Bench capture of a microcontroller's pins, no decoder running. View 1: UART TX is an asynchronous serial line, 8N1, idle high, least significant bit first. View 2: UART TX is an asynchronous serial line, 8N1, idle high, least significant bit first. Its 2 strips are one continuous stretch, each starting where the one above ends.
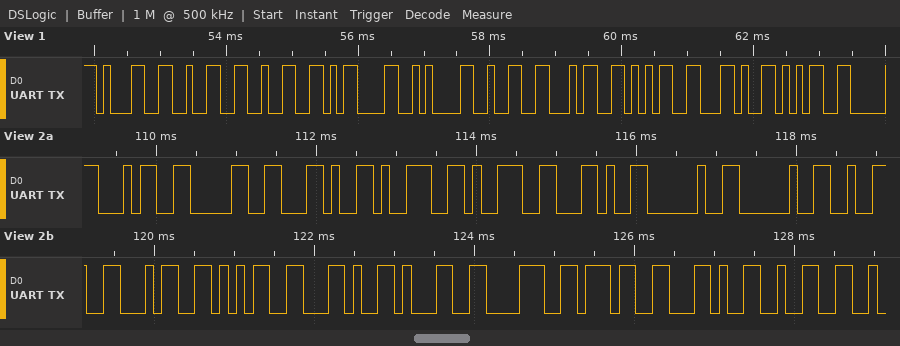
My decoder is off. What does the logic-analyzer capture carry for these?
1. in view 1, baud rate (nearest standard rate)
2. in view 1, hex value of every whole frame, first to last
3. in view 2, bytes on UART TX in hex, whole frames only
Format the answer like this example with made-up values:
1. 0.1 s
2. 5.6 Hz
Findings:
1. 9600 baud
2. 31 32 32 0D 0A 32 34 35 2C 35
3. 34 30 2C 39 39 2C 20 20 32 34 35 2C 31 38 37 2C 32
